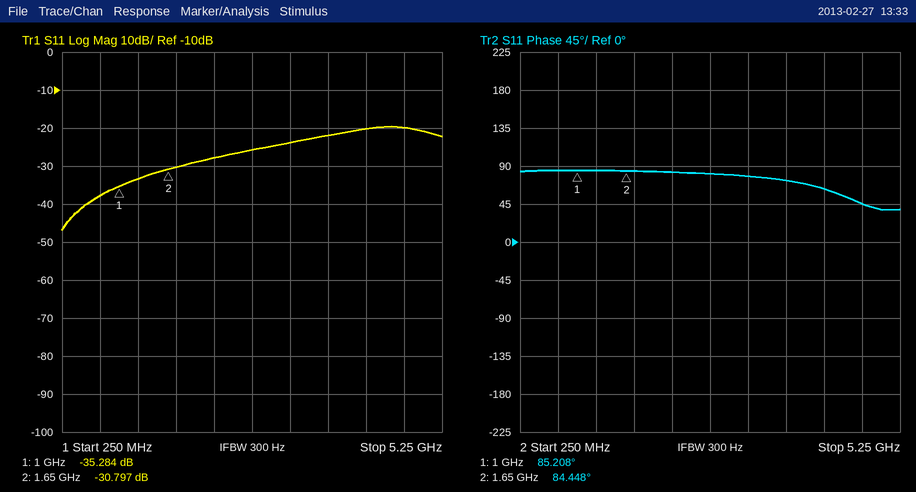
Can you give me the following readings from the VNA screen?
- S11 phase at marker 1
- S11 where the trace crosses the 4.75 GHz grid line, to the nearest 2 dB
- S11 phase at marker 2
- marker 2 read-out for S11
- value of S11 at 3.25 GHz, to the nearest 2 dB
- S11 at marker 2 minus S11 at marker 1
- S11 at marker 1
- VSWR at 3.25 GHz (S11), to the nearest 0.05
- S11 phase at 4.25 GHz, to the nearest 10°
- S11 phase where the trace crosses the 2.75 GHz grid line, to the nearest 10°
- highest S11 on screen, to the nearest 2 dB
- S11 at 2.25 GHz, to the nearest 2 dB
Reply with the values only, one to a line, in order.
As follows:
85.208°
-20 dB
84.448°
-30.797 dB
-24 dB
4.487 dB
-35.284 dB
1.15
60°
80°
-20 dB
-28 dB
